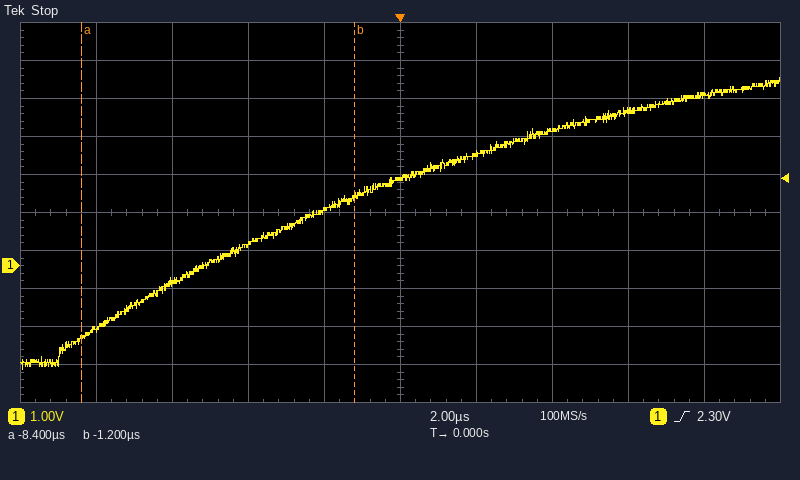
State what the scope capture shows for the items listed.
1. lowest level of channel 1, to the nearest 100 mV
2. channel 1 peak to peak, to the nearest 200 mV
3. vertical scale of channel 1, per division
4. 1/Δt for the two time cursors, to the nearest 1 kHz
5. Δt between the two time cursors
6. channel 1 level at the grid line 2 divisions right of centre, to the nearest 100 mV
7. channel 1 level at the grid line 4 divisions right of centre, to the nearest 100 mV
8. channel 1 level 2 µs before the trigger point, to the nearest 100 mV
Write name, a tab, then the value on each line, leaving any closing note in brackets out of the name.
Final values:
lowest level of channel 1, to the nearest 100 mV	-2.7 V
channel 1 peak to peak, to the nearest 200 mV	7.6 V
vertical scale of channel 1, per division	1 V
1/Δt for the two time cursors, to the nearest 1 kHz	139 kHz
Δt between the two time cursors	7.2 µs
channel 1 level at the grid line 2 divisions right of centre, to the nearest 100 mV	3.6 V
channel 1 level at the grid line 4 divisions right of centre, to the nearest 100 mV	4.5 V
channel 1 level 2 µs before the trigger point, to the nearest 100 mV	1.4 V
